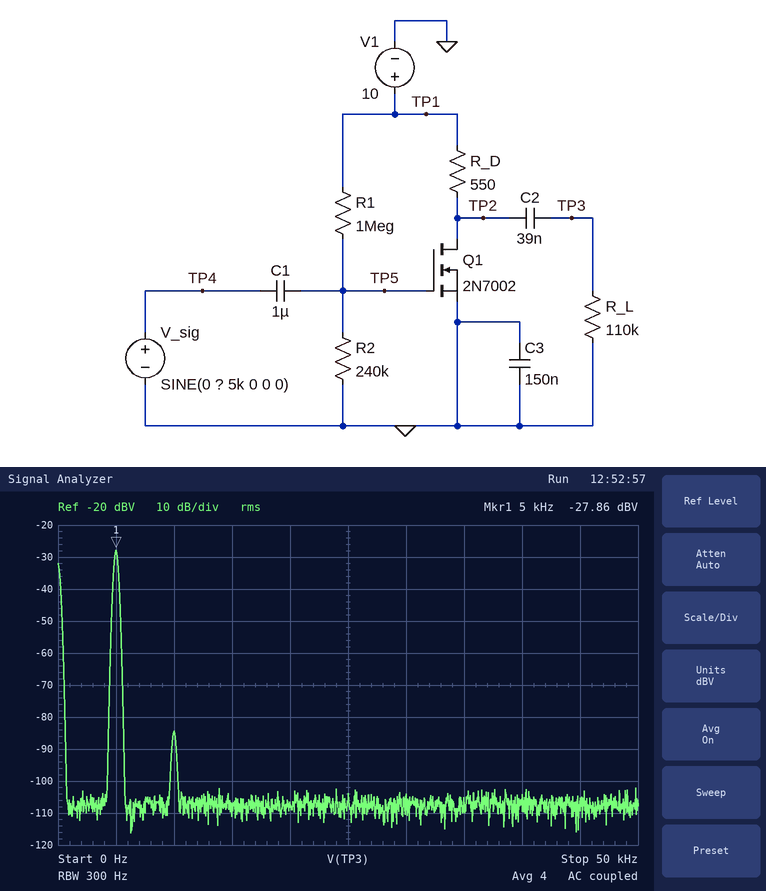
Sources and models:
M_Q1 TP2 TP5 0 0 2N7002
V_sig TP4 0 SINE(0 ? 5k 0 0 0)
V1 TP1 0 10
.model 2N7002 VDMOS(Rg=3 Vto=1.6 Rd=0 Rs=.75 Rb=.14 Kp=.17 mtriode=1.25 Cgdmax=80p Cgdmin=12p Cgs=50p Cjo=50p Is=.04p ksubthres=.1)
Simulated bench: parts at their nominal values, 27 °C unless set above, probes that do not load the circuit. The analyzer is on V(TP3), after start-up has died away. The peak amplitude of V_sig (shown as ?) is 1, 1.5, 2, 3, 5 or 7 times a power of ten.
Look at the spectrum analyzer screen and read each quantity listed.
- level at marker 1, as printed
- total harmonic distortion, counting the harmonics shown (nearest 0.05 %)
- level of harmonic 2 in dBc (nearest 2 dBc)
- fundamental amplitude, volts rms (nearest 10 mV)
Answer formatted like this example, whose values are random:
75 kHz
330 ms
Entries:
-27.86 dBV
0.15 %
-56 dBc
40 mV
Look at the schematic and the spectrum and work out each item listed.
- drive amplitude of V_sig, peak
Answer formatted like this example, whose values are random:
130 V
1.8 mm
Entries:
2 mV
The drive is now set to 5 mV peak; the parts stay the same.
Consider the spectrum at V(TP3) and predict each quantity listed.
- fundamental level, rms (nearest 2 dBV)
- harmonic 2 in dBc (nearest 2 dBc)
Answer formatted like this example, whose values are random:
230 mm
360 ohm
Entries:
-20 dBV
-48 dBc
